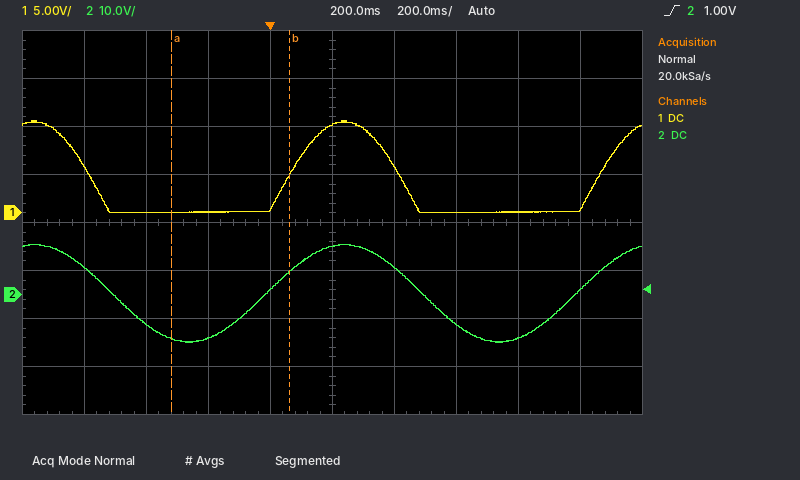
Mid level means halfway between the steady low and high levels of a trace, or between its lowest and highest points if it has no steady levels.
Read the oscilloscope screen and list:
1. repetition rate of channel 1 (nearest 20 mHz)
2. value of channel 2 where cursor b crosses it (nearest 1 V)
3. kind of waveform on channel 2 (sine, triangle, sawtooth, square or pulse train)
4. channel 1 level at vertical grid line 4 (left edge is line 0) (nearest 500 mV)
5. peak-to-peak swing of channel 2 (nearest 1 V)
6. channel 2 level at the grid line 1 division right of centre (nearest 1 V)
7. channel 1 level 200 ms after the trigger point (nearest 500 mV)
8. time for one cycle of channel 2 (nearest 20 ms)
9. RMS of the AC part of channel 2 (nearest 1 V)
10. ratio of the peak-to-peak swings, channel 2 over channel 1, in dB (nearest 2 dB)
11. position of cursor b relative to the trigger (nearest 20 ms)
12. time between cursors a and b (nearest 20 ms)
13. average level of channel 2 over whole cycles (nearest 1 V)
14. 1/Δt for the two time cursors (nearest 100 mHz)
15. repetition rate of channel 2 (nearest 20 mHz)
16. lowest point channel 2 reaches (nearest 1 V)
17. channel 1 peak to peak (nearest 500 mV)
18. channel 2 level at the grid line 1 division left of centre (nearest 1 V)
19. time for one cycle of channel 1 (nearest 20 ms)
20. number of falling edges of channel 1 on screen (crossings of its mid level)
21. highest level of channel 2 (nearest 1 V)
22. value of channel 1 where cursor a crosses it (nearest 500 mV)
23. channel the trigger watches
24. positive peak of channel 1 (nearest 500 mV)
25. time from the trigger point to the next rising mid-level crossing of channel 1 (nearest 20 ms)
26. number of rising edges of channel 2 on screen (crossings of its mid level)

1.00 Hz
5 V
sine
500 mV
20 V
6 V
9.0 V
1.00 s
7 V
6 dB
+60 ms
380 ms
0 V
2.6 Hz
1.00 Hz
-10 V
9.5 V
1 V
1.00 s
2
10 V
0.0 V
channel 2
9.5 V
80 ms
2
